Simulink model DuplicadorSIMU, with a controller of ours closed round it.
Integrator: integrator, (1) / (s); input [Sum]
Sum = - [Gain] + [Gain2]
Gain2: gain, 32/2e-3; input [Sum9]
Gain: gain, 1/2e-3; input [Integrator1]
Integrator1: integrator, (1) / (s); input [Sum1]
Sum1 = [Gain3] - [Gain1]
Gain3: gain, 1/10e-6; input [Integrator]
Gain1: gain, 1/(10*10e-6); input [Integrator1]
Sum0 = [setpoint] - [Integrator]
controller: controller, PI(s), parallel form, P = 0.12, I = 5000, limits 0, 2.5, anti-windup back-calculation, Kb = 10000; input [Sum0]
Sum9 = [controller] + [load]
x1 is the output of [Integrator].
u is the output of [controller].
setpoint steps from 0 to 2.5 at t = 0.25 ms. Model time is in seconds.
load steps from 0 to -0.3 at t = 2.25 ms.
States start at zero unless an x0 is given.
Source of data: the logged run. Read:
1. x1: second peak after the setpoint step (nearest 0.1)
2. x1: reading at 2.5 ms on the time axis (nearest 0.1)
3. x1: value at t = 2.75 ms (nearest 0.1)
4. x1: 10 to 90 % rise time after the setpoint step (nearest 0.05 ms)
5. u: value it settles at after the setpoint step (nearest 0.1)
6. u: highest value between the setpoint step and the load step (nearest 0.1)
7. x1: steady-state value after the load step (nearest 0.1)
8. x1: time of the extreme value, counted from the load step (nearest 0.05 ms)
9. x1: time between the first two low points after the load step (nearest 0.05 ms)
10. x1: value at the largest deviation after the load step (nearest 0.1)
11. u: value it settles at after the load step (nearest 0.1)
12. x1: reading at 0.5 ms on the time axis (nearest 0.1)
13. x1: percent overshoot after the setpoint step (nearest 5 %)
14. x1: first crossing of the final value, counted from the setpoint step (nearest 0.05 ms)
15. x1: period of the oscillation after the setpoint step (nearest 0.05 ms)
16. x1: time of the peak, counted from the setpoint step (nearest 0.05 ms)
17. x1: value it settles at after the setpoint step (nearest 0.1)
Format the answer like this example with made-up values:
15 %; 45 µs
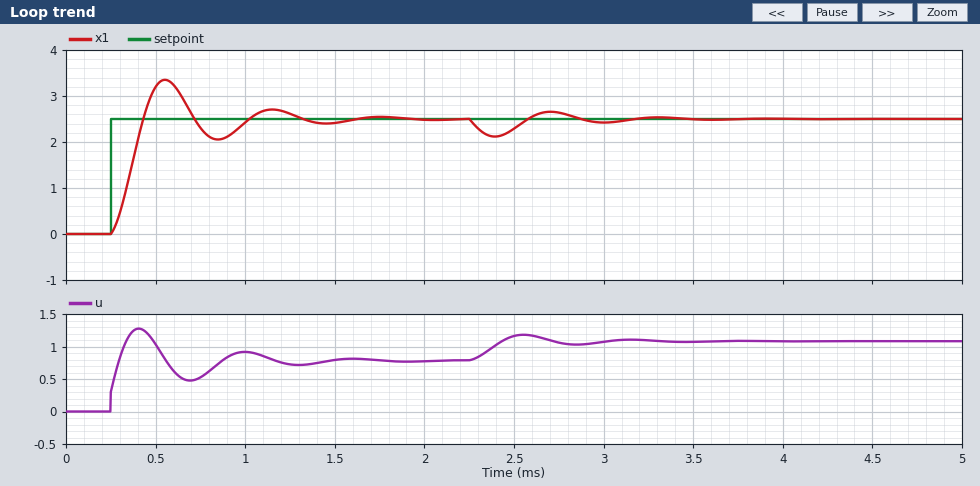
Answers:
2.7; 2.3; 2.6; 0.15 ms; 0.8; 1.3; 2.5; 0.15 ms; 0.60 ms; 2.1; 1.1; 3.2; 35 %; 0.20 ms; 0.60 ms; 0.30 ms; 2.5
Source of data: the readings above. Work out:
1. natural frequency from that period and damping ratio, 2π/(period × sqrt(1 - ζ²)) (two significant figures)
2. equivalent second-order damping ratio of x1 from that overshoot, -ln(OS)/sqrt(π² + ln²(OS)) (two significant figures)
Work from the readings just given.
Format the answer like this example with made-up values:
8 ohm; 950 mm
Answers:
11 rad/ms; 0.32
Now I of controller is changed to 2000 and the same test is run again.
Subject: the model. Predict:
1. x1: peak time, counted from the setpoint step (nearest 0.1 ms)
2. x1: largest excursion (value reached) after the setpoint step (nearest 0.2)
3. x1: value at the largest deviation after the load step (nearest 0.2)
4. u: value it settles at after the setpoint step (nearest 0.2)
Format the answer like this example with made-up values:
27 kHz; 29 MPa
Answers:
0.5 ms; 2.6; 2.0; 0.8
